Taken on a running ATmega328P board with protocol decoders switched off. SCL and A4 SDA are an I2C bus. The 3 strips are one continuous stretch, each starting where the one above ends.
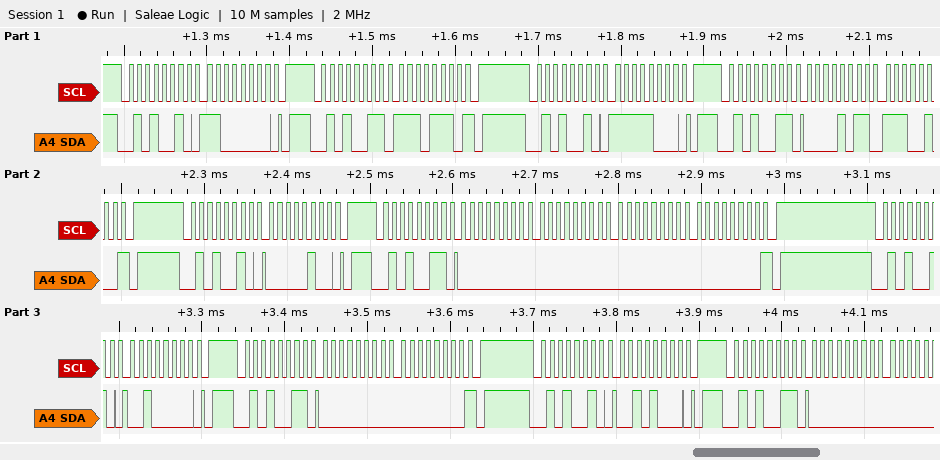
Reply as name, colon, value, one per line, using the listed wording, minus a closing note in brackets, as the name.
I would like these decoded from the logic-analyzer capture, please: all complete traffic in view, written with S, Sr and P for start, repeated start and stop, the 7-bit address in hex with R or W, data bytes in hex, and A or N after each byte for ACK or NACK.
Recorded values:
all complete traffic in view, written with S, Sr and P for start, repeated start and stop, the 7-bit address in hex with R or W, data bytes in hex, and A or N after each byte for ACK or NACK: S 29W A C0 A P S 29R A EE N P S 29W A F8 A P S 29R A 0B A E4 N P S 29W A 04 A P S 29R A 00 A 00 A 00 A 00 N P S 29W A 20 A P S 29R A 00 A 00 N P S 29W A 28 A P S 29R A 00 A
